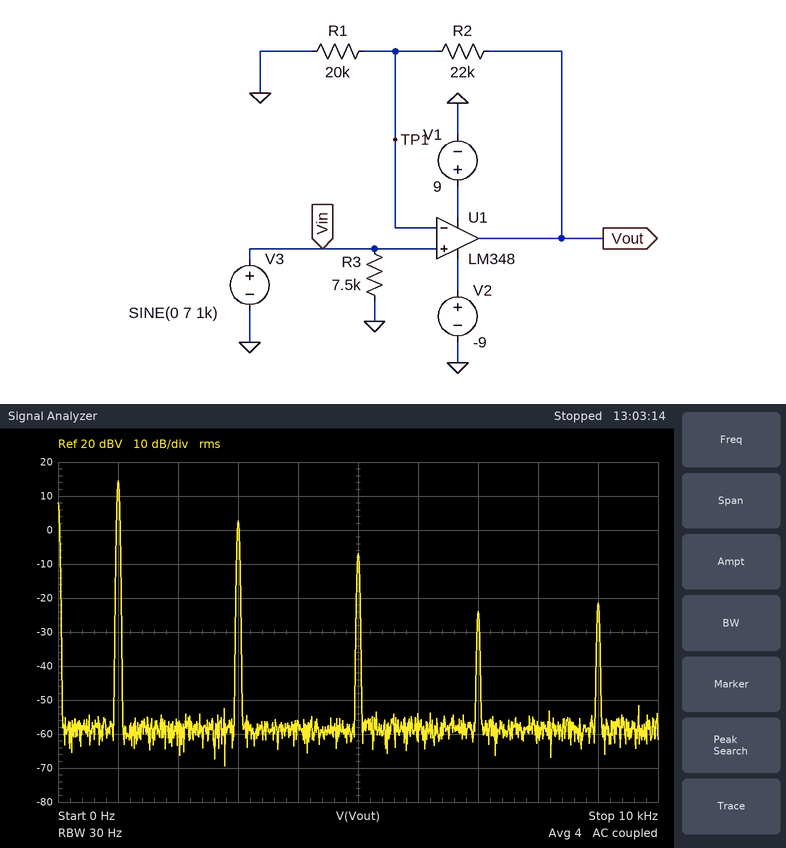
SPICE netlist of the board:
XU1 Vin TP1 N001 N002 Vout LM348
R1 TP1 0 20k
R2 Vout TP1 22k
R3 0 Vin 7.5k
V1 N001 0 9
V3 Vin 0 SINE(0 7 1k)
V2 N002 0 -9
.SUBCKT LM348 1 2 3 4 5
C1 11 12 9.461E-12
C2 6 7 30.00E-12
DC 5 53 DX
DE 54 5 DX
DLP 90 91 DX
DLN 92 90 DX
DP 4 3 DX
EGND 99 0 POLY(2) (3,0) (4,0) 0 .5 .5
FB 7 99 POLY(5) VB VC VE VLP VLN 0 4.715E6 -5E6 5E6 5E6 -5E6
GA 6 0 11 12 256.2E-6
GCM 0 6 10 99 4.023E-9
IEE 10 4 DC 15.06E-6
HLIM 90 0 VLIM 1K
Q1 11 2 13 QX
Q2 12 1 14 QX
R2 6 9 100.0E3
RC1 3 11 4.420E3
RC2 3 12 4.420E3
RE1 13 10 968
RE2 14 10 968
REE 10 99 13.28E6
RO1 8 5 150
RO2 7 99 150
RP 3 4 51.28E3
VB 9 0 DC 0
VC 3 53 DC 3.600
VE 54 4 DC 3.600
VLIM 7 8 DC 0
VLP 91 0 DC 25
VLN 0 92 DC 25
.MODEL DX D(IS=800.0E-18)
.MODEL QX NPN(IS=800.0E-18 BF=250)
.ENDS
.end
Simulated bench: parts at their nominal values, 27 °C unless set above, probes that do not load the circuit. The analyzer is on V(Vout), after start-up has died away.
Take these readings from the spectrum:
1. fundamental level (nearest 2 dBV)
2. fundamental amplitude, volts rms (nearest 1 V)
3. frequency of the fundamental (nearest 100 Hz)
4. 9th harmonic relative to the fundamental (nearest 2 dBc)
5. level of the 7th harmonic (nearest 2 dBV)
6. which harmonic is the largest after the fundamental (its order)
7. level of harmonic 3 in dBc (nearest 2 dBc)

14 dBV
5 V
1.0 kHz
-36 dBc
-24 dBV
3
-12 dBc
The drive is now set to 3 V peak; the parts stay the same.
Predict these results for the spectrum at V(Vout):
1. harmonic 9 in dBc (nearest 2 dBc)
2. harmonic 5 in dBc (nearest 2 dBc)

-46 dBc
-40 dBc
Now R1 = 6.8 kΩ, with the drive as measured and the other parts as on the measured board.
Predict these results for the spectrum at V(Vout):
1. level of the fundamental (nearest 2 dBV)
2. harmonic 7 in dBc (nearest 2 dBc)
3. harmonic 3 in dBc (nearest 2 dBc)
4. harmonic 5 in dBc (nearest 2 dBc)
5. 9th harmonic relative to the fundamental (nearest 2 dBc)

14 dBV
-20 dBc
-10 dBc
-16 dBc
-24 dBc
